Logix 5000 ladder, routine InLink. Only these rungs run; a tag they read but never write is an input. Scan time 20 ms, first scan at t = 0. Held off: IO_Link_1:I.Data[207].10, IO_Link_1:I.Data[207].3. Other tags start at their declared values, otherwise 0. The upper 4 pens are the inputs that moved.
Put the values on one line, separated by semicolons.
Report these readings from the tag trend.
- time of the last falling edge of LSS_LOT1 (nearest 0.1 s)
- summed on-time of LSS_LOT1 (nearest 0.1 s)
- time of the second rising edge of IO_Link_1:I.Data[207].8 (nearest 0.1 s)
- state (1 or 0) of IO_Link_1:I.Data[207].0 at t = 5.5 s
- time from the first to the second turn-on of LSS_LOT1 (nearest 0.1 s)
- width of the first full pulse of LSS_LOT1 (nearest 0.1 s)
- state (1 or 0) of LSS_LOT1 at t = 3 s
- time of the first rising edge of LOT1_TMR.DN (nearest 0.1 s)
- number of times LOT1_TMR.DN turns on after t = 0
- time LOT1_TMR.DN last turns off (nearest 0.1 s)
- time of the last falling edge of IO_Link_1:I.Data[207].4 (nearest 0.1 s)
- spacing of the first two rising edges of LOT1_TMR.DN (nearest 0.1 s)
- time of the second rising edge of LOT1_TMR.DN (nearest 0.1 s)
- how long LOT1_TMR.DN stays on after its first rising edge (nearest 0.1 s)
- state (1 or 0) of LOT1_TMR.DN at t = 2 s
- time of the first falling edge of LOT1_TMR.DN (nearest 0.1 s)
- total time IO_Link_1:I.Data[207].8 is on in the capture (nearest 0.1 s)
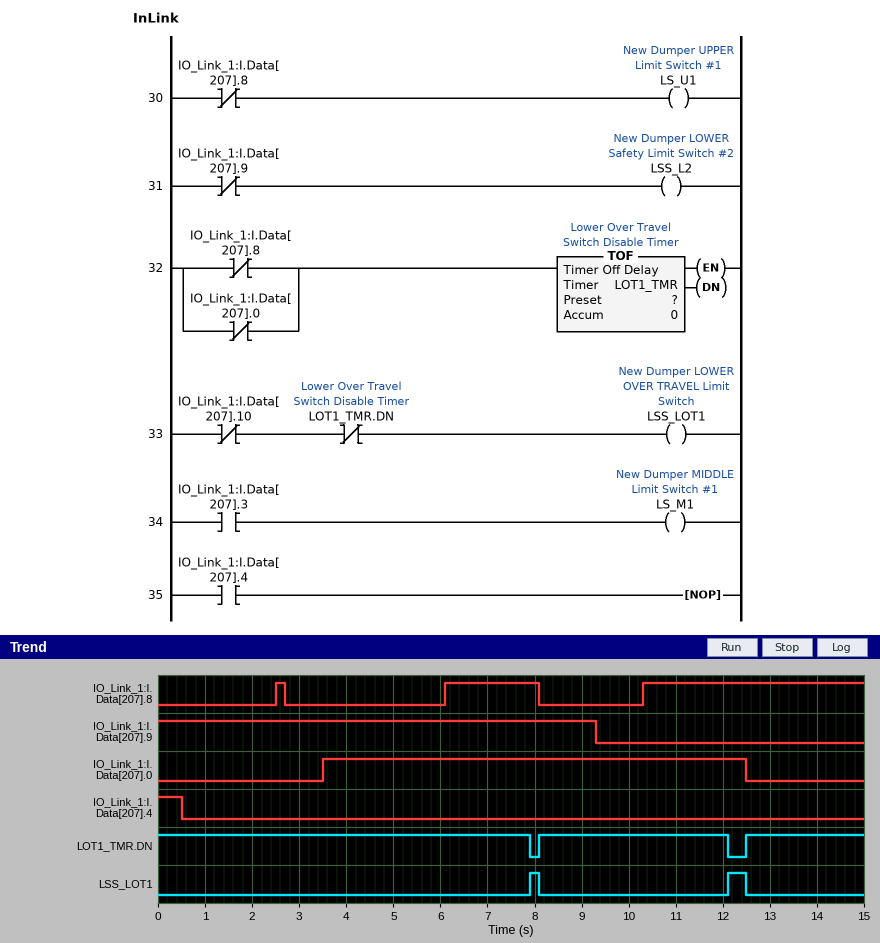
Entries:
12.5 s; 0.6 s; 6.1 s; 1; 4.2 s; 0.2 s; 0; 8.1 s; 2; 12.1 s; 0.5 s; 4.4 s; 12.5 s; 4.0 s; 1; 7.9 s; 6.9 s
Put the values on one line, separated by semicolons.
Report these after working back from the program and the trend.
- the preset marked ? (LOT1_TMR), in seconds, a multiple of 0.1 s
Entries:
1.8 s
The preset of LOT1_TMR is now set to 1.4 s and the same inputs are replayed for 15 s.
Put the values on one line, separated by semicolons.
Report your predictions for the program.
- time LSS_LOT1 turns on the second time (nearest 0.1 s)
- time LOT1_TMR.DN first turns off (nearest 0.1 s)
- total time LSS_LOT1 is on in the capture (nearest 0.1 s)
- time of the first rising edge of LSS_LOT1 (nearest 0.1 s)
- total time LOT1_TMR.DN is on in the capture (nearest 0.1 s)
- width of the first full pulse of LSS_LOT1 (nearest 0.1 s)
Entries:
11.7 s; 7.5 s; 1.4 s; 7.5 s; 13.6 s; 0.6 s
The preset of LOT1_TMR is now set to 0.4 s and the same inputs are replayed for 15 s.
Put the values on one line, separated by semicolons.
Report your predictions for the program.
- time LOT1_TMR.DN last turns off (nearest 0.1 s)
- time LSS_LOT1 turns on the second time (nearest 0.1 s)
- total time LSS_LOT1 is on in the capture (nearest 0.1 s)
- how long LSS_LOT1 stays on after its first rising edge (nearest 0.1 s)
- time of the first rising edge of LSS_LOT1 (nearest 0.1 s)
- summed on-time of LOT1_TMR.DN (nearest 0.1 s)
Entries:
10.7 s; 10.7 s; 3.4 s; 1.6 s; 6.5 s; 11.6 s
